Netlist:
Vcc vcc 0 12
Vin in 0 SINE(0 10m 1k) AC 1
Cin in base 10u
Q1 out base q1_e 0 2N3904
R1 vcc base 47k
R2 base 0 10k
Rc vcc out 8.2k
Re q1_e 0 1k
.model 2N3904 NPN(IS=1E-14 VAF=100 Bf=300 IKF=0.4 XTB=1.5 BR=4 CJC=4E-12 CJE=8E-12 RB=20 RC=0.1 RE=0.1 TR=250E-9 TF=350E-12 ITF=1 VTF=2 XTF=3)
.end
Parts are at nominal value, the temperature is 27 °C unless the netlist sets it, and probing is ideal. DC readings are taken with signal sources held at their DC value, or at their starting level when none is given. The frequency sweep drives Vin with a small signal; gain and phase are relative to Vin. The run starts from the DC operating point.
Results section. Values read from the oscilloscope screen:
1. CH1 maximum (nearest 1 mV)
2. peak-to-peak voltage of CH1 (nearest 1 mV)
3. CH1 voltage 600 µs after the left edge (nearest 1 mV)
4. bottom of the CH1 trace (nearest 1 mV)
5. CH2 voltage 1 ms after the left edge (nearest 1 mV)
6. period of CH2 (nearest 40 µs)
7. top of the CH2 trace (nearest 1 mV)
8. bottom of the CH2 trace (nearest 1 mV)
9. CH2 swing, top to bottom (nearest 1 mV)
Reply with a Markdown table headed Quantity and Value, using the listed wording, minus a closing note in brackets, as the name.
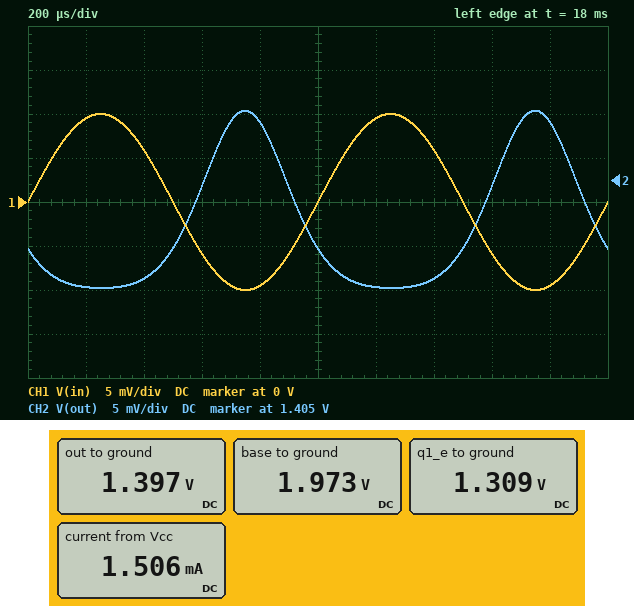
| Quantity | Value |
|---|---|
| CH1 maximum | 10 mV |
| peak-to-peak voltage of CH1 | 20 mV |
| CH1 voltage 600 µs after the left edge | -6 mV |
| bottom of the CH1 trace | -10 mV |
| CH2 voltage 1 ms after the left edge | 1.397 V |
| period of CH2 | 1.00 ms |
| top of the CH2 trace | 1.413 V |
| bottom of the CH2 trace | 1.393 V |
| CH2 swing, top to bottom | 20 mV |
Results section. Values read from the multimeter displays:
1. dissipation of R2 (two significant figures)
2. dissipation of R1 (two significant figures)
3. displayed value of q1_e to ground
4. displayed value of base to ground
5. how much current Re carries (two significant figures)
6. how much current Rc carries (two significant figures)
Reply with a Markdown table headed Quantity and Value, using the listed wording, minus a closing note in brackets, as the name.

| Quantity | Value |
|---|---|
| dissipation of R2 | 390 µW |
| dissipation of R1 | 2.1 mW |
| displayed value of q1_e to ground | 1.309 V |
| displayed value of base to ground | 1.973 V |
| how much current Re carries | 1.3 mA |
| how much current Rc carries | 1.3 mA |
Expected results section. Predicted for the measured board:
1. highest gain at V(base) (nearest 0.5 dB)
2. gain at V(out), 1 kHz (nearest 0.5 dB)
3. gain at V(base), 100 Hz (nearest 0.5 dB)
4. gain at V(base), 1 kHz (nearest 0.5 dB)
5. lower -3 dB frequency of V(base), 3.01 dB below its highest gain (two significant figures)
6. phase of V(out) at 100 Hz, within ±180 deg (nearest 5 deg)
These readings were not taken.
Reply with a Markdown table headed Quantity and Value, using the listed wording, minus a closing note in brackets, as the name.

| Quantity | Value |
|---|---|
| highest gain at V(base) | 0 dB |
| gain at V(out), 1 kHz | -2.0 dB |
| gain at V(base), 100 Hz | 0 dB |
| gain at V(base), 1 kHz | 0 dB |
| lower -3 dB frequency of V(base), 3.01 dB below its highest gain | 15 Hz |
| phase of V(out) at 100 Hz, within ±180 deg | -170 deg |
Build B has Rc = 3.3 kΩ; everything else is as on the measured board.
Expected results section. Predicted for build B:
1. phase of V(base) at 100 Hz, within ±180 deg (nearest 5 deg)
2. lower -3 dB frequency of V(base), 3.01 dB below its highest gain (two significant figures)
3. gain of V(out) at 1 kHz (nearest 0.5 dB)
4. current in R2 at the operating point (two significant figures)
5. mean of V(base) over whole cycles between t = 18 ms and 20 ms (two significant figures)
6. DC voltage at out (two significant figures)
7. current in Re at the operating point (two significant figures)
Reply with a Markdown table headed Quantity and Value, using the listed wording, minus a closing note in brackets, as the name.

| Quantity | Value |
|---|---|
| phase of V(base) at 100 Hz, within ±180 deg | 0 deg |
| lower -3 dB frequency of V(base), 3.01 dB below its highest gain | 2.0 Hz |
| gain of V(out) at 1 kHz | 10.0 dB |
| current in R2 at the operating point | 210 µA |
| mean of V(base) over whole cycles between t = 18 ms and 20 ms | 2.1 V |
| DC voltage at out | 7.4 V |
| current in Re at the operating point | 1.4 mA |
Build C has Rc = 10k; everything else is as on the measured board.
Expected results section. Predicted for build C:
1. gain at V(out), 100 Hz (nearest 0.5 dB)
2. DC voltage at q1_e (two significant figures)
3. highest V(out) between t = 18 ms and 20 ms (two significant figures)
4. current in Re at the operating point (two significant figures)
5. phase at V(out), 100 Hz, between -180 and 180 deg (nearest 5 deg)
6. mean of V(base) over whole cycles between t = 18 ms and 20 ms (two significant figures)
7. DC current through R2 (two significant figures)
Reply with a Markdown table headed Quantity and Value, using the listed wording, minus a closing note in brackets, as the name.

| Quantity | Value |
|---|---|
| gain at V(out), 100 Hz | -10.5 dB |
| DC voltage at q1_e | 1.1 V |
| highest V(out) between t = 18 ms and 20 ms | 1.2 V |
| current in Re at the operating point | 1.1 mA |
| phase at V(out), 100 Hz, between -180 and 180 deg | 10 deg |
| mean of V(base) over whole cycles between t = 18 ms and 20 ms | 1.8 V |
| DC current through R2 | 180 µA |
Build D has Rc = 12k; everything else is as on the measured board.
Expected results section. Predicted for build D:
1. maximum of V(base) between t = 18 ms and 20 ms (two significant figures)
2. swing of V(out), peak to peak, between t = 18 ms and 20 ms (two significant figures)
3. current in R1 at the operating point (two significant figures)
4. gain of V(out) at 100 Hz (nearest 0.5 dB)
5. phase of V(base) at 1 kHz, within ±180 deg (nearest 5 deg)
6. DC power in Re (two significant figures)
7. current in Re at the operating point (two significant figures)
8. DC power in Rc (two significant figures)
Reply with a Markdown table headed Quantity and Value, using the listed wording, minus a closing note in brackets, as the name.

| Quantity | Value |
|---|---|
| maximum of V(base) between t = 18 ms and 20 ms | 1.6 V |
| swing of V(out), peak to peak, between t = 18 ms and 20 ms | 11 mV |
| current in R1 at the operating point | 220 µA |
| gain of V(out) at 100 Hz | -5.5 dB |
| phase of V(base) at 1 kHz, within ±180 deg | 0 deg |
| DC power in Re | 950 µW |
| current in Re at the operating point | 970 µA |
| DC power in Rc | 10 mW |
